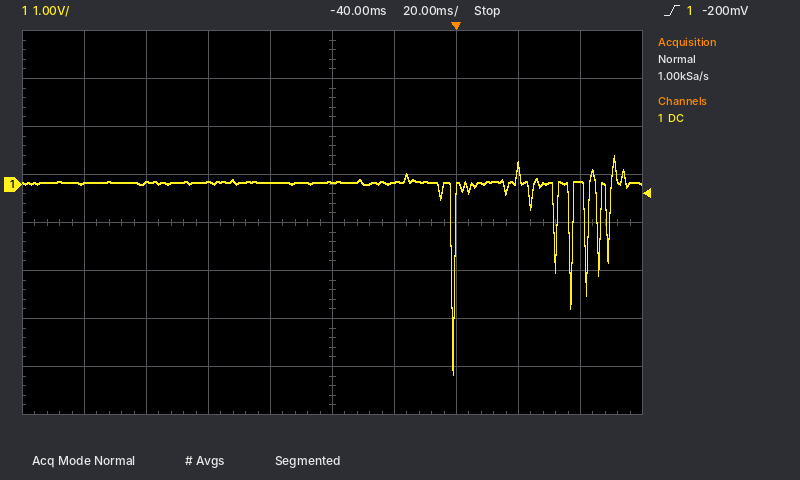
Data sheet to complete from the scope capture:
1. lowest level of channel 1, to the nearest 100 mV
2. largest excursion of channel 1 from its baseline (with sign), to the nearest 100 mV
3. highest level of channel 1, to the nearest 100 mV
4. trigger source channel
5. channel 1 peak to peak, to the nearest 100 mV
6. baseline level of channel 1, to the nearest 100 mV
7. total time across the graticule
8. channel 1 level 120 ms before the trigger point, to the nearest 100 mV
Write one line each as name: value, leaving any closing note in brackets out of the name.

lowest level of channel 1, to the nearest 100 mV: -4.0 V
largest excursion of channel 1 from its baseline (with sign), to the nearest 100 mV: -4.0 V
highest level of channel 1, to the nearest 100 mV: 600 mV
trigger source channel: channel 1
channel 1 peak to peak, to the nearest 100 mV: 4.6 V
baseline level of channel 1, to the nearest 100 mV: 0.0 V
total time across the graticule: 200 ms
channel 1 level 120 ms before the trigger point, to the nearest 100 mV: 0.0 V
